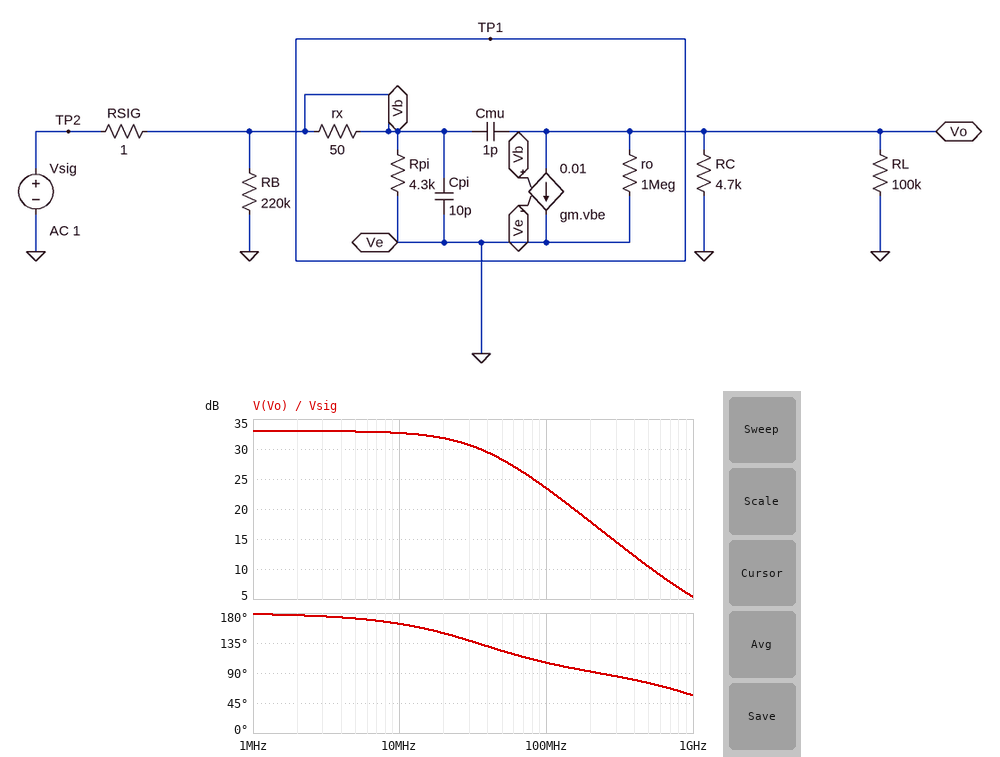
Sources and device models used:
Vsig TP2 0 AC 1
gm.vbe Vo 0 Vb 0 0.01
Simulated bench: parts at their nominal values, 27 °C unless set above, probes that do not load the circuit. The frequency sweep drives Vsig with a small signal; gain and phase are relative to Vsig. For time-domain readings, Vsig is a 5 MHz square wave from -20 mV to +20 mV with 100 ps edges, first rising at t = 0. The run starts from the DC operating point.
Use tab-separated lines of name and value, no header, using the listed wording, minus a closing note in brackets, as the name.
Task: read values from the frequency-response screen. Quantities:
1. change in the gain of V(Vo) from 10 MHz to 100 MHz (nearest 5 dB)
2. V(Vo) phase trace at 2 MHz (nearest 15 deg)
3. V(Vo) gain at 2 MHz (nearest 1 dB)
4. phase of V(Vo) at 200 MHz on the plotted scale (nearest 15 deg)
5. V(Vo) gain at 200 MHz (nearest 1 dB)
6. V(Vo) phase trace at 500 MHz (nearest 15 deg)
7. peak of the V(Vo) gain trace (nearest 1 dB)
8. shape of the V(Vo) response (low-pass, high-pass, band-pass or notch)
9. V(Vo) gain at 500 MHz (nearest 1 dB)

change in the gain of V(Vo) from 10 MHz to 100 MHz	-10 dB
V(Vo) phase trace at 2 MHz	180 deg
V(Vo) gain at 2 MHz	33 dB
phase of V(Vo) at 200 MHz on the plotted scale	90 deg
V(Vo) gain at 200 MHz	18 dB
V(Vo) phase trace at 500 MHz	75 deg
peak of the V(Vo) gain trace	33 dB
shape of the V(Vo) response	low-pass
V(Vo) gain at 500 MHz	10 dB
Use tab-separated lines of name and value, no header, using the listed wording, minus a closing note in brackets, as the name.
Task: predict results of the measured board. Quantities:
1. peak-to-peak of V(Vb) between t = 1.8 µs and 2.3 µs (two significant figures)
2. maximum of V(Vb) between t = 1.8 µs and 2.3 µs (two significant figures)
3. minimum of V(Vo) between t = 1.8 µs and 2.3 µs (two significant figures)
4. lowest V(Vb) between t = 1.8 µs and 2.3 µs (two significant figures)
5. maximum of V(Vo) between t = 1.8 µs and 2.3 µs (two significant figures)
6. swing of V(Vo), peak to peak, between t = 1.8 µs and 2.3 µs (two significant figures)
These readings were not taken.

peak-to-peak of V(Vb) between t = 1.8 µs and 2.3 µs	40 mV
maximum of V(Vb) between t = 1.8 µs and 2.3 µs	20 mV
minimum of V(Vo) between t = 1.8 µs and 2.3 µs	-910 mV
lowest V(Vb) between t = 1.8 µs and 2.3 µs	-20 mV
maximum of V(Vo) between t = 1.8 µs and 2.3 µs	910 mV
swing of V(Vo), peak to peak, between t = 1.8 µs and 2.3 µs	1.8 V
